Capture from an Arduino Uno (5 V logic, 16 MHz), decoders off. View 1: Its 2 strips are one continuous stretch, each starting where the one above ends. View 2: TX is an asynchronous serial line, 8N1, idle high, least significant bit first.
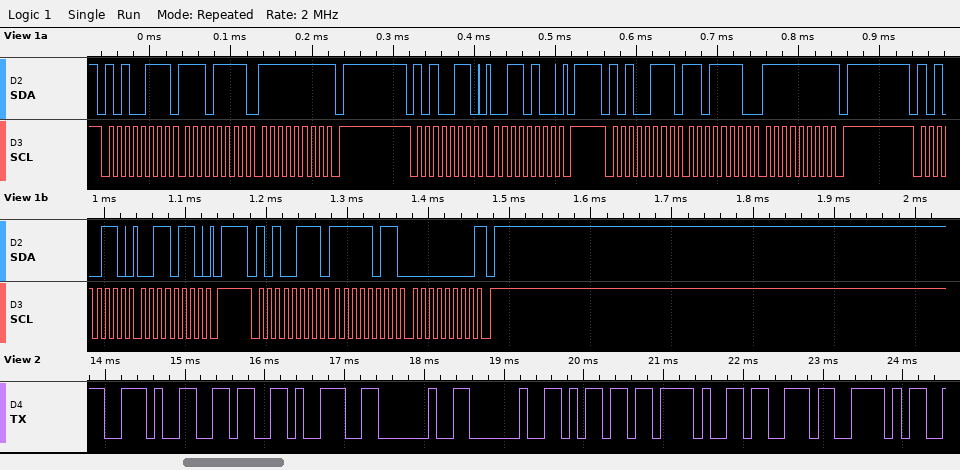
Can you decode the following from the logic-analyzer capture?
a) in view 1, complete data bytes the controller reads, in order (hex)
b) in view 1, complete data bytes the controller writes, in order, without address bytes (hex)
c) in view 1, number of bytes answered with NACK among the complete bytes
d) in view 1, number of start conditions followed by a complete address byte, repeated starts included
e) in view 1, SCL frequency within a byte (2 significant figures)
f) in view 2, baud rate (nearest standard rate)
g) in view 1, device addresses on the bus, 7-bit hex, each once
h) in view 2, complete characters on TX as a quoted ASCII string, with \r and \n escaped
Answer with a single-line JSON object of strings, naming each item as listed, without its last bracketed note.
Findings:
{"in view 1, complete data bytes the controller reads, in order": "EF FF DE FF FB 00", "in view 1, complete data bytes the controller writes, in order, without address bytes": "34 36", "in view 1, number of bytes answered with NACK among the complete bytes": "3", "in view 1, number of start conditions followed by a complete address byte, repeated starts included": "5", "in view 1, SCL frequency within a byte": "100 kHz", "in view 2, baud rate": "9600 baud", "in view 1, device addresses on the bus, 7-bit hex, each once": "0x53", "in view 2, complete characters on TX as a quoted ASCII string, with \\r and \\n escaped": "\".69  m/s^\""}
